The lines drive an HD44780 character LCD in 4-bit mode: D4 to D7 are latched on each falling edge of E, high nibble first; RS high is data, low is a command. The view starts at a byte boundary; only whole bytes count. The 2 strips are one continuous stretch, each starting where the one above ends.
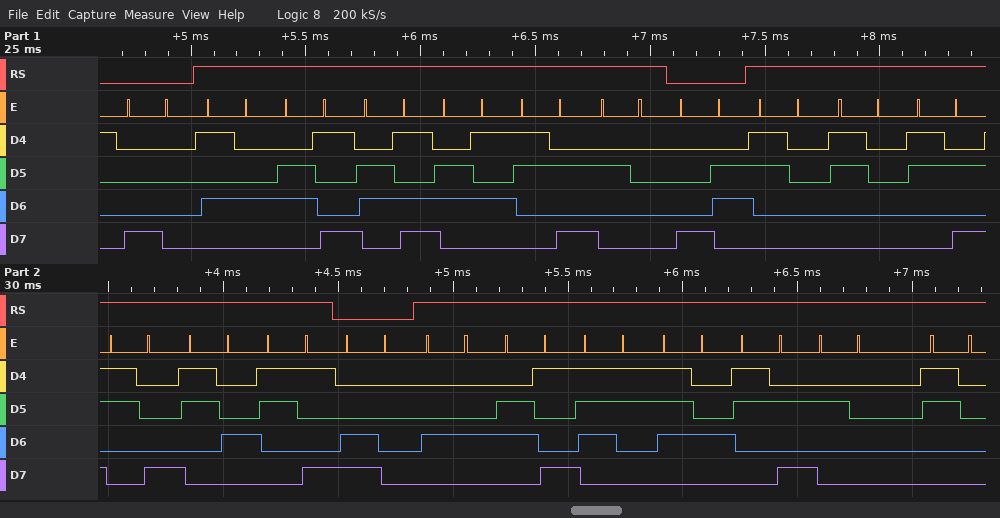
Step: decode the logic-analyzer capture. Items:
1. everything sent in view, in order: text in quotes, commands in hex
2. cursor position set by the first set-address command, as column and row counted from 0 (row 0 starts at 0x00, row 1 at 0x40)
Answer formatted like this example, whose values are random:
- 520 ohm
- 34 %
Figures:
- 0x80 "Time: " 0x86 "00:849" 0xC0 "Dist: 0"
- column 0, row 0
